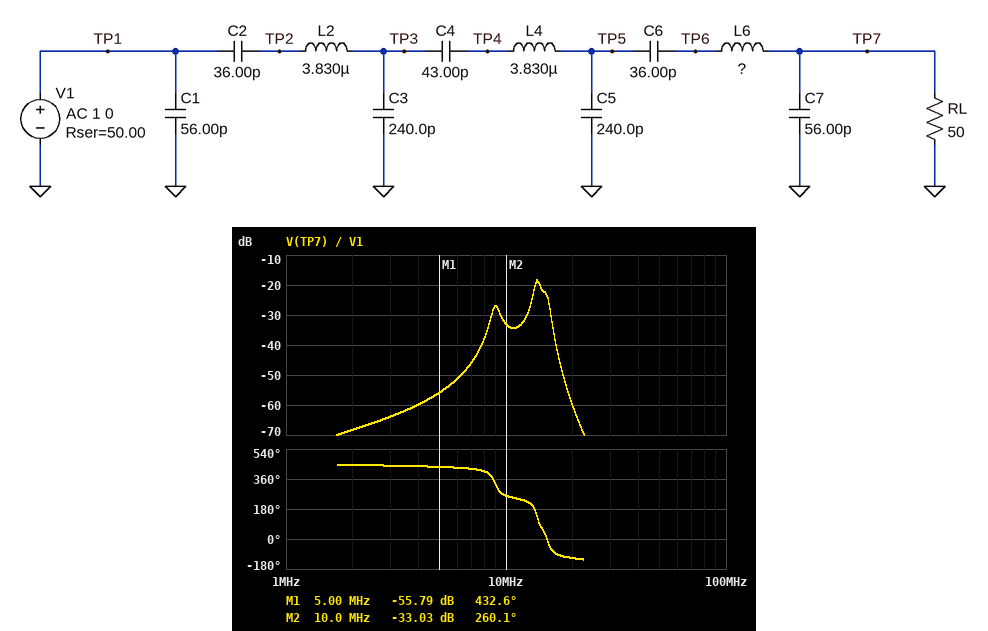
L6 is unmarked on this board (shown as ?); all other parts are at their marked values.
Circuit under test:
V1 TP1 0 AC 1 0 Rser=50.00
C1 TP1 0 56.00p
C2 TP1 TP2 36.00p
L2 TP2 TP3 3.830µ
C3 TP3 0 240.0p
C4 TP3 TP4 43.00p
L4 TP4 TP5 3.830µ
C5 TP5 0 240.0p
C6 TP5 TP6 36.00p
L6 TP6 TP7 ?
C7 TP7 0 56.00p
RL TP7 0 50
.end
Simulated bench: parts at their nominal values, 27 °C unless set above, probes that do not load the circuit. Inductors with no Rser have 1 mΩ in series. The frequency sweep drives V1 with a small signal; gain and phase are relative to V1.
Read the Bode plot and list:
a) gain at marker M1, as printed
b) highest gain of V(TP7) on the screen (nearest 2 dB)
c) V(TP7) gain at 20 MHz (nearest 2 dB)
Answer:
-55.79 dB
-18 dB
-60 dB
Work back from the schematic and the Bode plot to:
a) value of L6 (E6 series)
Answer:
10 µH
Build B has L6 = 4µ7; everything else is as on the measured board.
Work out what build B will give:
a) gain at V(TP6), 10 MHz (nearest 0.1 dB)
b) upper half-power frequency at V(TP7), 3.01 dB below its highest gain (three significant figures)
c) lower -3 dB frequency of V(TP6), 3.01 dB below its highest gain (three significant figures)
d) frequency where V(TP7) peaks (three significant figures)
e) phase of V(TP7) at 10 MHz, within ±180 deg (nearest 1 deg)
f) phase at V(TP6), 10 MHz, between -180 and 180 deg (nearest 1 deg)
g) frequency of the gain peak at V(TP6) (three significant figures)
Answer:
-21.2 dB
15.5 MHz
13.1 MHz
14.1 MHz
46 deg
136 deg
14.2 MHz
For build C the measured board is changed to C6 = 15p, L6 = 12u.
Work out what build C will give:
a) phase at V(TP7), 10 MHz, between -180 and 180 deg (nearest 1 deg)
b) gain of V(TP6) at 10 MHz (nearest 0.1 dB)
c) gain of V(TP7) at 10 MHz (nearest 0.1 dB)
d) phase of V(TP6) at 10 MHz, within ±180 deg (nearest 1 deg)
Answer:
52 deg
-17.9 dB
-41.5 dB
148 deg
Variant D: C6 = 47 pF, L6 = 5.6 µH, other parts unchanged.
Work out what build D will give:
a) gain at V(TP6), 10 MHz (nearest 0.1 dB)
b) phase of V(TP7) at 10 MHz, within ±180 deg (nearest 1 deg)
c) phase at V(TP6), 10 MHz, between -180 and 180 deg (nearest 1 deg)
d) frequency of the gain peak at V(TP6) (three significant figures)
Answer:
-9.6 dB
11 deg
103 deg
14.0 MHz
